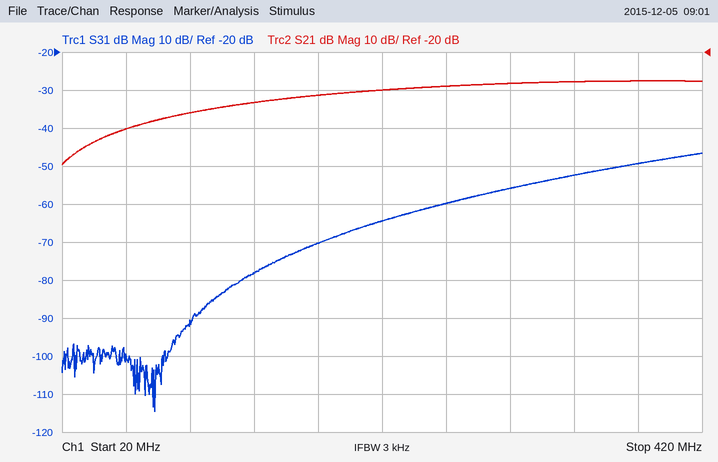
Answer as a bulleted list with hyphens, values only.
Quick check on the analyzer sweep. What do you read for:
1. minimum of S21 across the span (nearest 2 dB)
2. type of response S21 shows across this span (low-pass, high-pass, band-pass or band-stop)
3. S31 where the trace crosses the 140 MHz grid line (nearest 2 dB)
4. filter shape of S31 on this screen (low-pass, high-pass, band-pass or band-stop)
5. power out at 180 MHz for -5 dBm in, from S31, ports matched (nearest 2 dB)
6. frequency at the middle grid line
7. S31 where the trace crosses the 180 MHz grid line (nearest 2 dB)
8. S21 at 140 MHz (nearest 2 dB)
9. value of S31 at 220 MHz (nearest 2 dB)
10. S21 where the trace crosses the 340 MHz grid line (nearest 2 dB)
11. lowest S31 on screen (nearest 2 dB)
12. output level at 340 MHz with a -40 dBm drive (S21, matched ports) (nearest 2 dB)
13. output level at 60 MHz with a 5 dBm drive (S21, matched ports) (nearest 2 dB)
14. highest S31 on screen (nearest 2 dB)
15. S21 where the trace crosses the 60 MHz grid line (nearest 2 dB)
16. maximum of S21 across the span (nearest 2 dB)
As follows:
- -50 dB
- high-pass
- -78 dB
- high-pass
- -76 dBm
- 220 MHz
- -70 dB
- -34 dB
- -64 dB
- -28 dB
- -114 dB
- -68 dBm
- -36 dBm
- -46 dB
- -40 dB
- -28 dB
